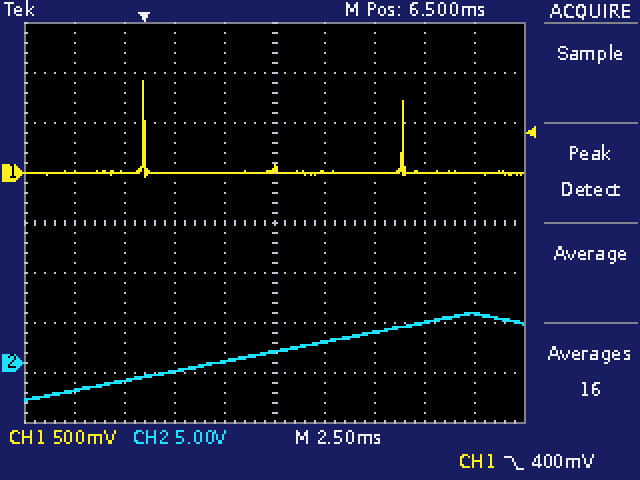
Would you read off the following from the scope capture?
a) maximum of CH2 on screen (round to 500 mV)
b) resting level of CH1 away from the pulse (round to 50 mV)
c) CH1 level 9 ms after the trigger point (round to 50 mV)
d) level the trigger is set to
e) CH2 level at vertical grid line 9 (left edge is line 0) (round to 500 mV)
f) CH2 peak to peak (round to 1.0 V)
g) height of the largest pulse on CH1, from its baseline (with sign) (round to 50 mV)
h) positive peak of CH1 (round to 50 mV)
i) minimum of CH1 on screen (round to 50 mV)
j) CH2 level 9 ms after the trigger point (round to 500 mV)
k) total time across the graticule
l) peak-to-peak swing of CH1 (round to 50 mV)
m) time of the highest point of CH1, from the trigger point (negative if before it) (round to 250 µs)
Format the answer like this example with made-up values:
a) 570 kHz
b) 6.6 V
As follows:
a) 5.0 V
b) 0 mV
c) 0 mV
d) 400 mV
e) 5.0 V
f) 9.0 V
g) +900 mV
h) 900 mV
i) -50 mV
j) 2.0 V
k) 25 ms
l) 950 mV
m) 0.00 ms
